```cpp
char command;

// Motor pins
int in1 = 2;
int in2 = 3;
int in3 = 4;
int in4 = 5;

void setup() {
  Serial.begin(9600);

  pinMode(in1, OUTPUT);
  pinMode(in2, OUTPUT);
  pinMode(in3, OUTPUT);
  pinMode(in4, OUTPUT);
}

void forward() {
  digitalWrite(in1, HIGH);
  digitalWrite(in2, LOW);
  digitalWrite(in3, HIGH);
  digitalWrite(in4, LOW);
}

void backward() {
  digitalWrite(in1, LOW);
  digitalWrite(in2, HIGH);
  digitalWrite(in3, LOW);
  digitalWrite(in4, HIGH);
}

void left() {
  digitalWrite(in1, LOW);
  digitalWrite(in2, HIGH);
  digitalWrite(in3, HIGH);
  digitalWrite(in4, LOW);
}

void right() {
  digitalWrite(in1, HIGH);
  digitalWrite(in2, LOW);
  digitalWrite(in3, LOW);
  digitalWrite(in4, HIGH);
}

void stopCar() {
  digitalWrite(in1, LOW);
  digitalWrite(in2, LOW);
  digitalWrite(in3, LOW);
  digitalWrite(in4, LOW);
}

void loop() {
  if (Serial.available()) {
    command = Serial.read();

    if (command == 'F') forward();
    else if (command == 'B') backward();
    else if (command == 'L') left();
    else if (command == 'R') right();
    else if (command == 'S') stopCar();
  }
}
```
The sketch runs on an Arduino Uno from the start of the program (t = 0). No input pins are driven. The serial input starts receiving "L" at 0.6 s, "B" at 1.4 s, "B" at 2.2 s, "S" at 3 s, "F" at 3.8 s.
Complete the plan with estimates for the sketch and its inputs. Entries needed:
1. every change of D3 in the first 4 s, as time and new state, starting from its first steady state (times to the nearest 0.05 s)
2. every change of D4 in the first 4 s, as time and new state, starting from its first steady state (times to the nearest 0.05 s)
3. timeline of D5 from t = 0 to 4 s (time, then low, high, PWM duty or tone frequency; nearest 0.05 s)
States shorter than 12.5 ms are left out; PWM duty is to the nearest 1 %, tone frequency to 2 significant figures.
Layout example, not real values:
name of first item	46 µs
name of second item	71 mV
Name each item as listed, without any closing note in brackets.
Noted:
every change of D3 in the first 4 s, as time and new state, starting from its first steady state	0 s low; 0.6 s high; 3 s low
every change of D4 in the first 4 s, as time and new state, starting from its first steady state	0 s low; 0.6 s high; 1.4 s low; 3.8 s high
timeline of D5 from t = 0 to 4 s	0 s low; 1.4 s high; 3 s low
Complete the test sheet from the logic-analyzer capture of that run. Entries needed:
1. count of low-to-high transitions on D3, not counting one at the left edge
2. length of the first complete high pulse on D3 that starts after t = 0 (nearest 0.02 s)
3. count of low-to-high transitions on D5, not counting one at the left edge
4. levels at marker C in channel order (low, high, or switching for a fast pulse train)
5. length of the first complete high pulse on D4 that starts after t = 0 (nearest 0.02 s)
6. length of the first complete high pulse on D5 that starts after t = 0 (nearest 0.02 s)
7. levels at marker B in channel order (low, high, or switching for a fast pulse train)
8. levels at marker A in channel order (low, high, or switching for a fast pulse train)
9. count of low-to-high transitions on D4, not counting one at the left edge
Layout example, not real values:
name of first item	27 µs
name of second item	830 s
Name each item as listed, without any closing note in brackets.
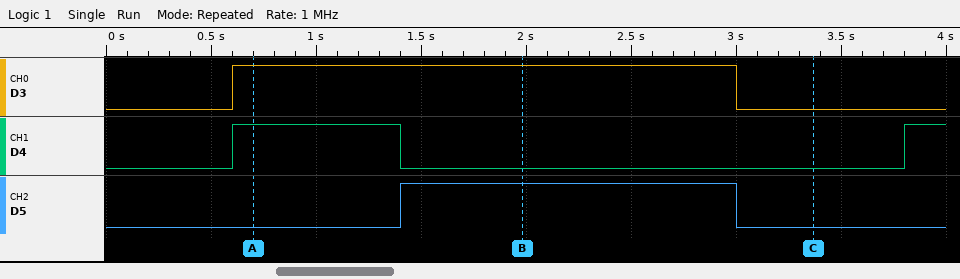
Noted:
count of low-to-high transitions on D3, not counting one at the left edge	1
length of the first complete high pulse on D3 that starts after t = 0	2.40 s
count of low-to-high transitions on D5, not counting one at the left edge	1
levels at marker C in channel order	D3 low, D4 low, D5 low
length of the first complete high pulse on D4 that starts after t = 0	0.80 s
length of the first complete high pulse on D5 that starts after t = 0	1.60 s
levels at marker B in channel order	D3 high, D4 low, D5 high
levels at marker A in channel order	D3 high, D4 high, D5 low
count of low-to-high transitions on D4, not counting one at the left edge	2
